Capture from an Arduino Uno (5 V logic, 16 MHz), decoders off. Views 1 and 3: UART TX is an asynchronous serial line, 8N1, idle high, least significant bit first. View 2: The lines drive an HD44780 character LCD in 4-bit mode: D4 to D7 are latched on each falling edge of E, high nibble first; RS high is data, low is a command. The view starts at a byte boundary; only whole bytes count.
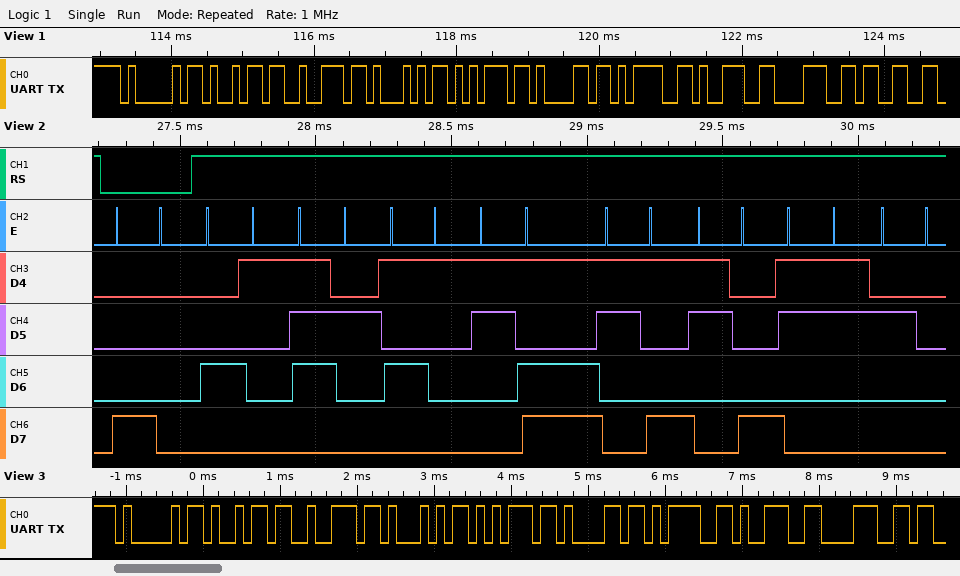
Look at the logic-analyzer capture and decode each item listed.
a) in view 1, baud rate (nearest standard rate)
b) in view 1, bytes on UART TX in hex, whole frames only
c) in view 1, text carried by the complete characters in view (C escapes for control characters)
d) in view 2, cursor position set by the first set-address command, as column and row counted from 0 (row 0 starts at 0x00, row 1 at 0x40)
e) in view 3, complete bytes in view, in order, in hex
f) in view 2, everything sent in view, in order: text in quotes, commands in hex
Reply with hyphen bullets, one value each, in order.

- 9600 baud
- 41 69 72 51 75 61 3D 39 38 33
- "AirQua=983"
- column 0, row 0
- 41 69 72 51 75 61 3D 39 38
- 0x80 "ArQ=983 "
